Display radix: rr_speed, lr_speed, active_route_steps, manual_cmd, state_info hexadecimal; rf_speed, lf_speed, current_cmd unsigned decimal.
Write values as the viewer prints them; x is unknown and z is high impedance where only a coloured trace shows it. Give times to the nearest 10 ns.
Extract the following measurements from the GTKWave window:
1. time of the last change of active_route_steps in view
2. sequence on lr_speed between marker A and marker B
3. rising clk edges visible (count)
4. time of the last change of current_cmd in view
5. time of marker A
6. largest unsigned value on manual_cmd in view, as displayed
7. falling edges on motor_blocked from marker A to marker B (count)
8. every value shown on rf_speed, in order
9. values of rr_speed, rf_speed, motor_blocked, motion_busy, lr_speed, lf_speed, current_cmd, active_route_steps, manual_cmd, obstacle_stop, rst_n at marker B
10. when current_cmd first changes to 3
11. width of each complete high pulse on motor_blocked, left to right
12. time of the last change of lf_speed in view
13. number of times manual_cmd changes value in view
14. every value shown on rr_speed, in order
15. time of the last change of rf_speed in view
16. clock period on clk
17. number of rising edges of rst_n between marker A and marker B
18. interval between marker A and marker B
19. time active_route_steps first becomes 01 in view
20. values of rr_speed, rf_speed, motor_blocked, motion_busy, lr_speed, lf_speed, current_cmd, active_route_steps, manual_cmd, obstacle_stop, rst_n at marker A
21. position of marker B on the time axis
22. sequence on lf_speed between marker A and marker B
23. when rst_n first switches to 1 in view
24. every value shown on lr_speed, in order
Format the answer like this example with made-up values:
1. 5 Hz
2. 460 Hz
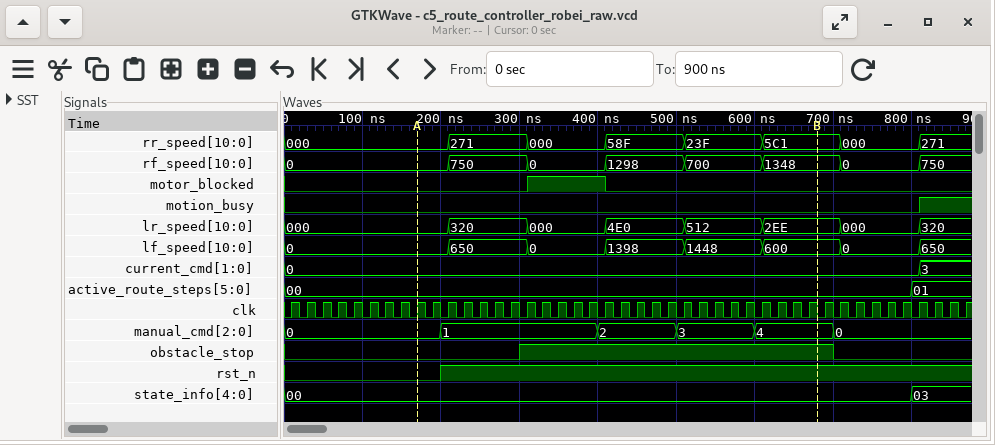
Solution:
1. 800 ns
2. 000, 320, 000, 4E0, 512, 2EE
3. 44
4. 810 ns
5. 170 ns
6. 4
7. 1
8. 0, 750, 0, 1298, 700, 1348, 0, 750
9. rr_speed=5C1, rf_speed=1348, motor_blocked=0, motion_busy=0, lr_speed=2EE, lf_speed=600, current_cmd=0, active_route_steps=00, manual_cmd=4, obstacle_stop=1, rst_n=1
10. 810 ns
11. 100 ns
12. 810 ns
13. 5
14. 000, 271, 000, 58F, 23F, 5C1, 000, 271
15. 810 ns
16. 20 ns
17. 1
18. 510 ns
19. 800 ns
20. rr_speed=000, rf_speed=0, motor_blocked=0, motion_busy=0, lr_speed=000, lf_speed=0, current_cmd=0, active_route_steps=00, manual_cmd=0, obstacle_stop=0, rst_n=0
21. 680 ns
22. 0, 650, 0, 1398, 1448, 600
23. 200 ns
24. 000, 320, 000, 4E0, 512, 2EE, 000, 320
